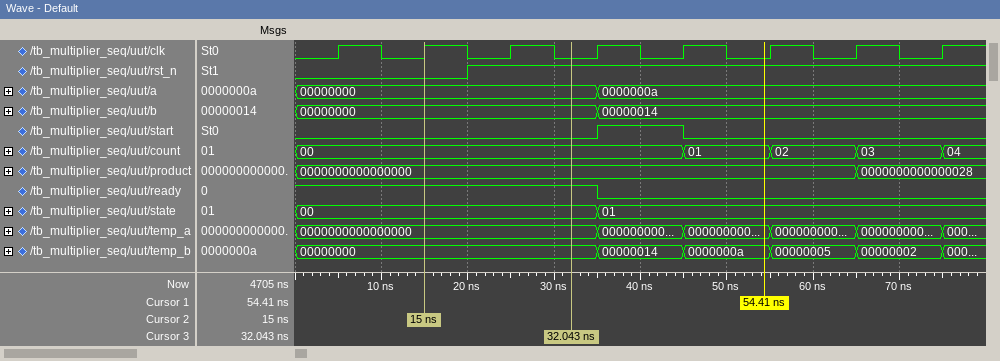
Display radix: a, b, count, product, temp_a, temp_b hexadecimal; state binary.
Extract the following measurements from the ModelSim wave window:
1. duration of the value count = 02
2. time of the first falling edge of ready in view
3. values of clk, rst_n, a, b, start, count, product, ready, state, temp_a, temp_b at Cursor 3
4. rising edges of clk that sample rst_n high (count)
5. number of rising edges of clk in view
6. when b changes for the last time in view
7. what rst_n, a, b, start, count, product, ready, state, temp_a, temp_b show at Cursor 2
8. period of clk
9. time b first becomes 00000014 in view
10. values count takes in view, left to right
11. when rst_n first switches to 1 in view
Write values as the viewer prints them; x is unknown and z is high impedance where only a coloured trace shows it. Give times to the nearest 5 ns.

10 ns
35 ns
clk=0, rst_n=1, a=00000000, b=00000000, start=0, count=00, product=0000000000000000, ready=1, state=00, temp_a=0000000000000000, temp_b=00000000
6
8
35 ns
rst_n=0, a=00000000, b=00000000, start=0, count=00, product=0000000000000000, ready=1, state=00, temp_a=0000000000000000, temp_b=00000000
10 ns
35 ns
00, 01, 02, 03, 04
20 ns
